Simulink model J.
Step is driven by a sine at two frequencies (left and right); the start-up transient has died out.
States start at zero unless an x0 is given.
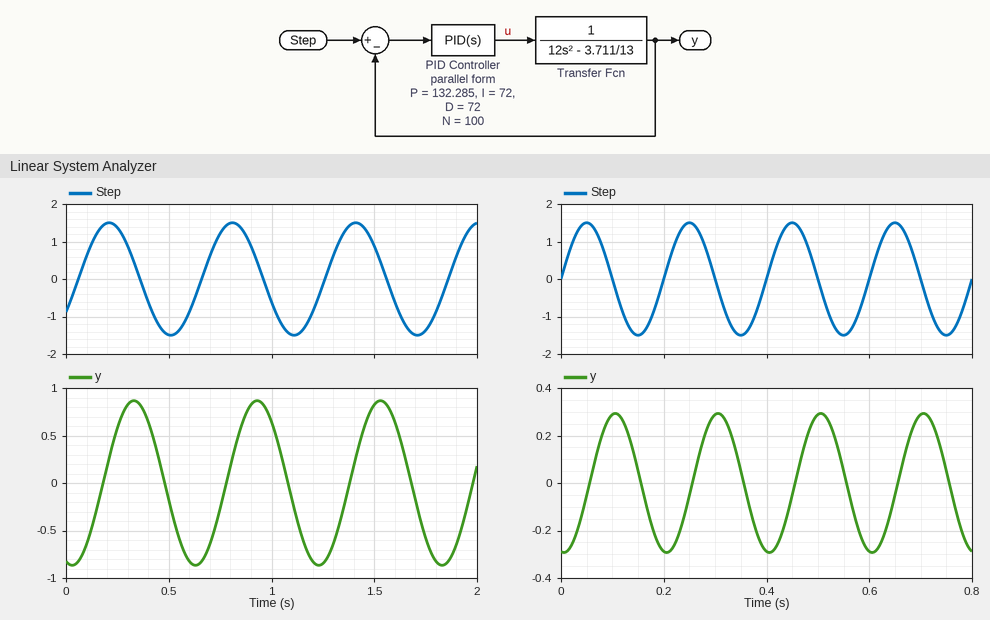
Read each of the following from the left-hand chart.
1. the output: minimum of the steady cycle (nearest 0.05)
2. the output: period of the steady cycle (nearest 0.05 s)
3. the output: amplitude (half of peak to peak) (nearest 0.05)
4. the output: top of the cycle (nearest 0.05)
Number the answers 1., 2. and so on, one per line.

1. -0.85
2. 0.60 s
3. 0.85
4. 0.85
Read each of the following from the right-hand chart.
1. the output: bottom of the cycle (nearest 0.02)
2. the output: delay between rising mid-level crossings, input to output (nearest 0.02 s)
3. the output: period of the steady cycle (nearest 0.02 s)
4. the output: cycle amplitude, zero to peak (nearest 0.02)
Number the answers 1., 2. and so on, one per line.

1. -0.30
2. 0.06 s
3. 0.20 s
4. 0.30
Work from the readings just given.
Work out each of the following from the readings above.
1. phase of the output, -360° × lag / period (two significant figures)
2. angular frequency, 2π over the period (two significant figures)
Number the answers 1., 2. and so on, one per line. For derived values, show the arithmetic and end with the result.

1. -360 × 0.06 / 0.2 = -110°
2. 2π / 0.2 = 31 rad/s
